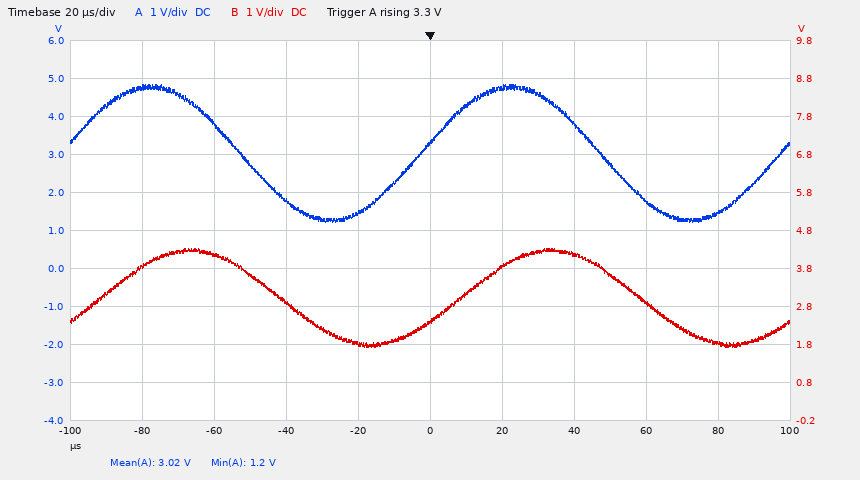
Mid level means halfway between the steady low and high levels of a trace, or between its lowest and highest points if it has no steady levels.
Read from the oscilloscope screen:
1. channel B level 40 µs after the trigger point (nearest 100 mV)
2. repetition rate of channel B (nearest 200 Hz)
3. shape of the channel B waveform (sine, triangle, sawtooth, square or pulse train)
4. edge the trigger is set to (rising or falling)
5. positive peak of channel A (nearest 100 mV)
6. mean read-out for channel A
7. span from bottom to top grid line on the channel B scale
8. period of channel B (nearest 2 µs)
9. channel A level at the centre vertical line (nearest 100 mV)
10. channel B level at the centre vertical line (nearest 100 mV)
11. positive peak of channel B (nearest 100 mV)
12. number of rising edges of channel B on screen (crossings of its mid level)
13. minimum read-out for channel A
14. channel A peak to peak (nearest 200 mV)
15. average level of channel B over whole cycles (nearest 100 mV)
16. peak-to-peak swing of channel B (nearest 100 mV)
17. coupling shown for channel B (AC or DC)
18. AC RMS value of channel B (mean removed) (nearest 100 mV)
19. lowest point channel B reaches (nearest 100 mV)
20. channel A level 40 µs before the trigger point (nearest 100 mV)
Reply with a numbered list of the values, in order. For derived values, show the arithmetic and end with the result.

1. 4.2 V
2. 1 / 100 µs ≈ 10.0 kHz
3. sine
4. rising
5. 4.8 V
6. 3.02 V
7. 10 V
8. 100 µs
9. 3.3 V
10. 2.4 V
11. 4.3 V
12. 2
13. 1.2 V
14. 3.6 V
15. (4.3 V + (1.7 V)) / 2 ≈ 3.0 V
16. 4.3 V − (1.7 V) = 2.6 V
17. DC
18. 2.6 V / (2√2) ≈ 919 mV, so 900 mV to the nearest 100 mV
19. 1.7 V
20. 1.8 V
